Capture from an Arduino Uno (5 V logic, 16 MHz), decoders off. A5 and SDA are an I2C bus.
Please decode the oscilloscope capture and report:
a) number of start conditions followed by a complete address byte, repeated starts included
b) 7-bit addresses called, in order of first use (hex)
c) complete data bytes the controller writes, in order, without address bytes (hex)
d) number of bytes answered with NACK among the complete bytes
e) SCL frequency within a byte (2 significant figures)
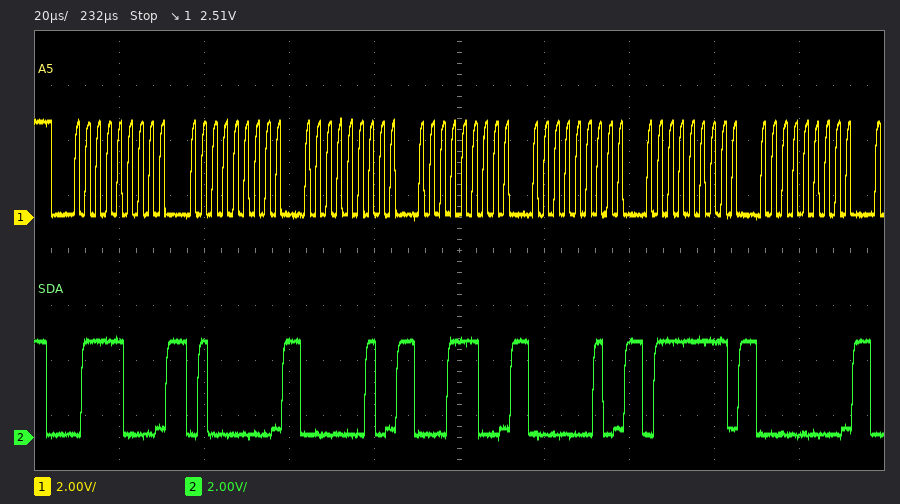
1
0x3C
40 02 1C 02 7F 00
0
400 kHz
